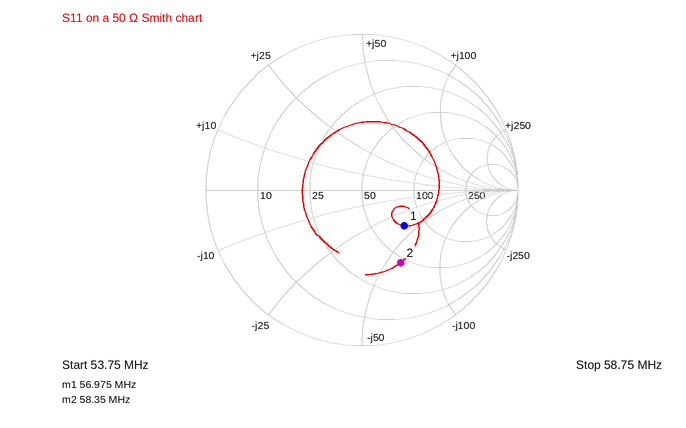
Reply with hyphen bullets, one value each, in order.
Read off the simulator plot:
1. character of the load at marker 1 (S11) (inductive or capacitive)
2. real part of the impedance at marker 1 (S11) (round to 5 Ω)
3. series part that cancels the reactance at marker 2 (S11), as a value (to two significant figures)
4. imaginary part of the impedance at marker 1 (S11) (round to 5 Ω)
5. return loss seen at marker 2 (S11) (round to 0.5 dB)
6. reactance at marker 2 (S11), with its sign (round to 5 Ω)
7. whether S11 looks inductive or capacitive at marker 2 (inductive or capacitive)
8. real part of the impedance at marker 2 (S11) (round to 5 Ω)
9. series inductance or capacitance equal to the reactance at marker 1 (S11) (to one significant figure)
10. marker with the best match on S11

- capacitive
- 75 Ω
- 160 nH
- -40 Ω
- 5.5 dB
- -60 Ω
- capacitive
- 45 Ω
- 70 pF
- marker 1
